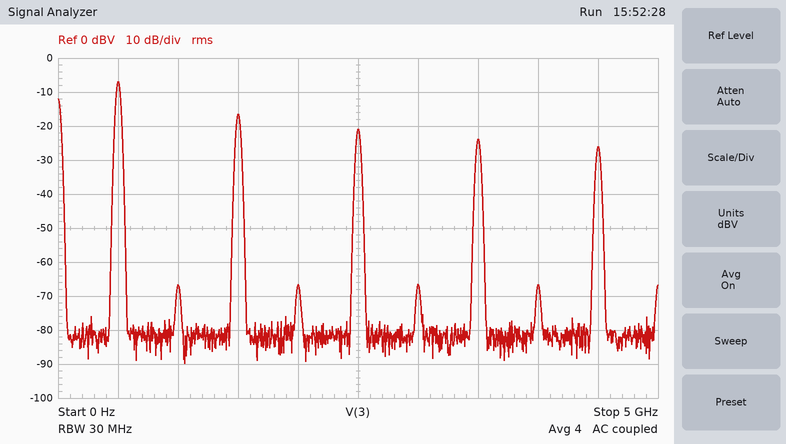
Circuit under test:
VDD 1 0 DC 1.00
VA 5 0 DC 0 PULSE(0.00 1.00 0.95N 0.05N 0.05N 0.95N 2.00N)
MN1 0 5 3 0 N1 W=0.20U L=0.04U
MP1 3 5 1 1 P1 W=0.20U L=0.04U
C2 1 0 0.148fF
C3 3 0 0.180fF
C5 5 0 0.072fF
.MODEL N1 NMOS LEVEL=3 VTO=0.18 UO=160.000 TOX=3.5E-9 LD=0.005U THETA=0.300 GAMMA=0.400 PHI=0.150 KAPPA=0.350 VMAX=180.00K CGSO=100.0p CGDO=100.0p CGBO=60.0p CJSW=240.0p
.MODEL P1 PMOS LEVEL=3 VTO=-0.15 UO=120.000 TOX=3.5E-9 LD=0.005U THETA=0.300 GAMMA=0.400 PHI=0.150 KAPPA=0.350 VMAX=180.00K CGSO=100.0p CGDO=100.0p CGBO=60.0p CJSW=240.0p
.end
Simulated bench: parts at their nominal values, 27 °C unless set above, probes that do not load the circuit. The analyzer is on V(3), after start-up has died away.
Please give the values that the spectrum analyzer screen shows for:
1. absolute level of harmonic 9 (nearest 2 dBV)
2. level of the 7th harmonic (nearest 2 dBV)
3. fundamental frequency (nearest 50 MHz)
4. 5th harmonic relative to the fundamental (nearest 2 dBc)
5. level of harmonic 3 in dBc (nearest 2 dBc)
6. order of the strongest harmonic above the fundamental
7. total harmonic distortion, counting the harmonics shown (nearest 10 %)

-26 dBV
-24 dBV
500 MHz
-14 dBc
-10 dBc
3
40 %
